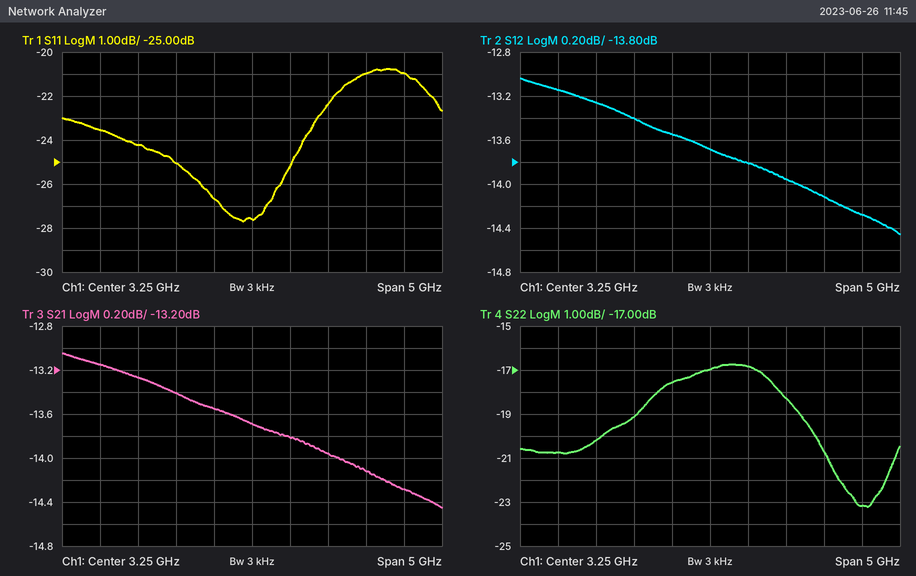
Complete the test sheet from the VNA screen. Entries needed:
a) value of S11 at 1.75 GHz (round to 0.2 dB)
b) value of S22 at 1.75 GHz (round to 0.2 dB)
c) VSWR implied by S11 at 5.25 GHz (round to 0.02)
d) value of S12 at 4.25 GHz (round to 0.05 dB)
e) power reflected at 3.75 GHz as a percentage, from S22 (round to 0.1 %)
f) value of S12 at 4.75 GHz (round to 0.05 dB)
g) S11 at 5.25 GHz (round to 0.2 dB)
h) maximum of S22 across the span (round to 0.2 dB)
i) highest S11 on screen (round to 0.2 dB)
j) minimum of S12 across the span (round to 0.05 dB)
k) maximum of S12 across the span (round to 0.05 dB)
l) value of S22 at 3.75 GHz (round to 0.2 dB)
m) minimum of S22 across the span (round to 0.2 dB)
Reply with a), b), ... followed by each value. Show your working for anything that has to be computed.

a) -24.2 dB
b) -20.2 dB
c) |Γ| = 10^(-21/20) = 0.0891; VSWR = (1 + 0.0891)/(1 − 0.0891) ≈ 1.20
d) -13.95 dB
e) 10^(-16.8/10) ≈ 2.1 %
f) -14.10 dB
g) -21.0 dB
h) -16.8 dB
i) -20.8 dB
j) -14.45 dB
k) -13.05 dB
l) -16.8 dB
m) -23.2 dB
